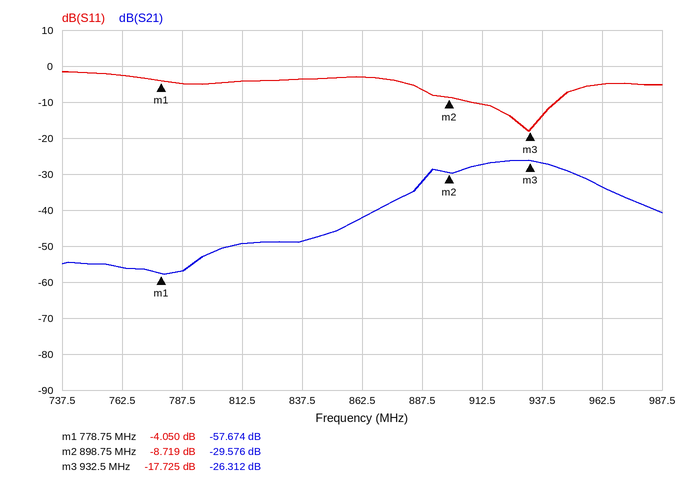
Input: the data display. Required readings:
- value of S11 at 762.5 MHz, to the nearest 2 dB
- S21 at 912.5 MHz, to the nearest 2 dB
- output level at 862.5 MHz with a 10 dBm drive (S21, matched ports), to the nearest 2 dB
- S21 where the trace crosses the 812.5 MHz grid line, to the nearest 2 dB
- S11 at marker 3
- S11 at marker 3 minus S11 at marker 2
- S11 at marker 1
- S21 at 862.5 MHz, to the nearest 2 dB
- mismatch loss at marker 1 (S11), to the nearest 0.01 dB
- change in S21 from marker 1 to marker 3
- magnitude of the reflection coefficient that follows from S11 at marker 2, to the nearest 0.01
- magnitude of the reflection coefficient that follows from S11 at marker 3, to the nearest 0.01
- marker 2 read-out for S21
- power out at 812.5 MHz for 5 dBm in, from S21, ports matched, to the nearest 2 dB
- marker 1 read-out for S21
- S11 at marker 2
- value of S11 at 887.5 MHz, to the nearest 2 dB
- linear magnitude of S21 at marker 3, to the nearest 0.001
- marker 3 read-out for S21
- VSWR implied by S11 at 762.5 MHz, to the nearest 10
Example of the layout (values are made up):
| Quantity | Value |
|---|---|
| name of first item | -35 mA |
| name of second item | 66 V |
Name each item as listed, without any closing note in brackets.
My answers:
| Quantity | Value |
|---|---|
| value of S11 at 762.5 MHz, to the nearest 2 dB | -2 dB |
| S21 at 912.5 MHz, to the nearest 2 dB | -28 dB |
| output level at 862.5 MHz with a 10 dBm drive (S21, matched ports), to the nearest 2 dB | -32 dBm |
| S21 where the trace crosses the 812.5 MHz grid line, to the nearest 2 dB | -50 dB |
| S11 at marker 3 | -17.725 dB |
| S11 at marker 3 minus S11 at marker 2 | -9.006 dB |
| S11 at marker 1 | -4.050 dB |
| S21 at 862.5 MHz, to the nearest 2 dB | -42 dB |
| mismatch loss at marker 1 (S11), to the nearest 0.01 dB | 2.17 dB |
| change in S21 from marker 1 to marker 3 | 31.362 dB |
| magnitude of the reflection coefficient that follows from S11 at marker 2, to the nearest 0.01 | 0.37 |
| magnitude of the reflection coefficient that follows from S11 at marker 3, to the nearest 0.01 | 0.13 |
| marker 2 read-out for S21 | -29.576 dB |
| power out at 812.5 MHz for 5 dBm in, from S21, ports matched, to the nearest 2 dB | -44 dBm |
| marker 1 read-out for S21 | -57.674 dB |
| S11 at marker 2 | -8.719 dB |
| value of S11 at 887.5 MHz, to the nearest 2 dB | -6 dB |
| linear magnitude of S21 at marker 3, to the nearest 0.001 | 0.048 |
| marker 3 read-out for S21 | -26.312 dB |
| VSWR implied by S11 at 762.5 MHz, to the nearest 10 | 10 |
